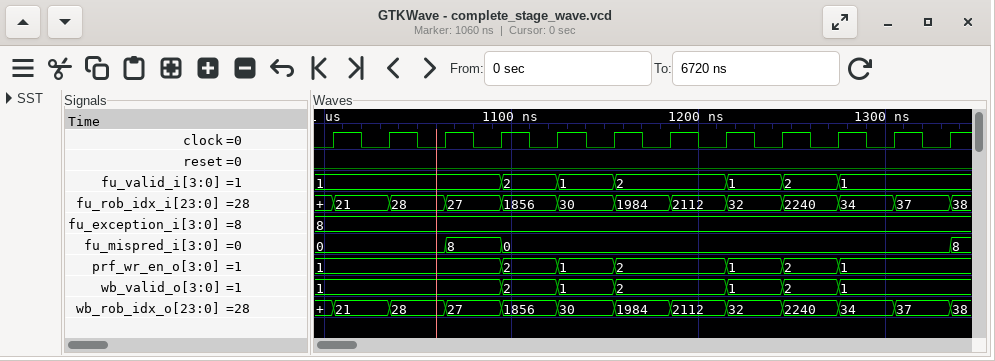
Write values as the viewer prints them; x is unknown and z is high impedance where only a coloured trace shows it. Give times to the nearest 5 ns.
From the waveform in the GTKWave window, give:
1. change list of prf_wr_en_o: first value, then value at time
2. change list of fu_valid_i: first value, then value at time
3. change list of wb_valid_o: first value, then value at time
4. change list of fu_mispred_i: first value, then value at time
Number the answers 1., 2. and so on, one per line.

1. 1, 2 at 1095 ns, 1 at 1125 ns, 2 at 1155 ns, 1 at 1215 ns, 2 at 1245 ns, 1 at 1275 ns
2. 1, 2 at 1095 ns, 1 at 1125 ns, 2 at 1155 ns, 1 at 1215 ns, 2 at 1245 ns, 1 at 1275 ns
3. 1, 2 at 1095 ns, 1 at 1125 ns, 2 at 1155 ns, 1 at 1215 ns, 2 at 1245 ns, 1 at 1275 ns
4. 0, 8 at 1065 ns, 0 at 1095 ns, 8 at 1335 ns
